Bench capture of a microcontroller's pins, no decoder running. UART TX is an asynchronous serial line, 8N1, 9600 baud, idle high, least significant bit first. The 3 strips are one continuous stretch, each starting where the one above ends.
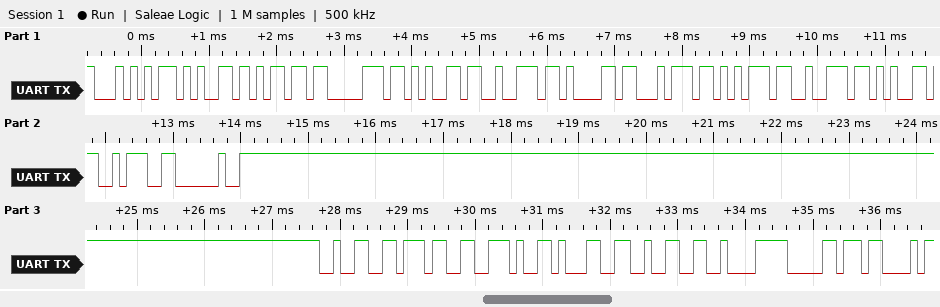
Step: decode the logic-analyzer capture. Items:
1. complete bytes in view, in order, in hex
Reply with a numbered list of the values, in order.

1. 0x54 0x65 0x6D 0x70 0x65 0x72 0x61 0x74 0x75 0x72 0x65 0x3A 0x20 0x32 0x37 0x2E 0x31 0x32 0xC2 0xB0 0x43
